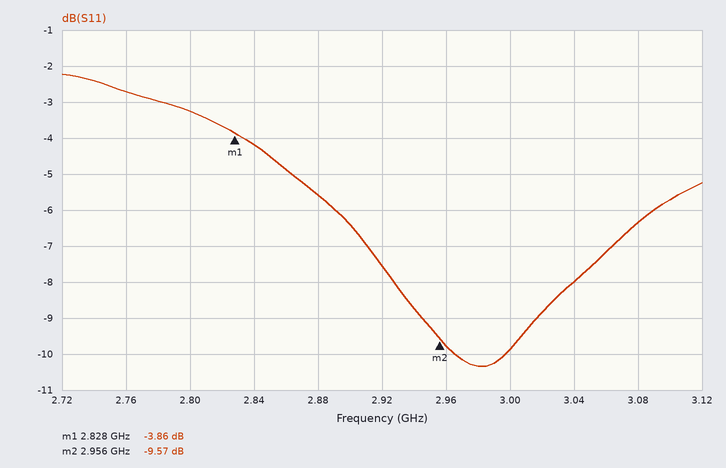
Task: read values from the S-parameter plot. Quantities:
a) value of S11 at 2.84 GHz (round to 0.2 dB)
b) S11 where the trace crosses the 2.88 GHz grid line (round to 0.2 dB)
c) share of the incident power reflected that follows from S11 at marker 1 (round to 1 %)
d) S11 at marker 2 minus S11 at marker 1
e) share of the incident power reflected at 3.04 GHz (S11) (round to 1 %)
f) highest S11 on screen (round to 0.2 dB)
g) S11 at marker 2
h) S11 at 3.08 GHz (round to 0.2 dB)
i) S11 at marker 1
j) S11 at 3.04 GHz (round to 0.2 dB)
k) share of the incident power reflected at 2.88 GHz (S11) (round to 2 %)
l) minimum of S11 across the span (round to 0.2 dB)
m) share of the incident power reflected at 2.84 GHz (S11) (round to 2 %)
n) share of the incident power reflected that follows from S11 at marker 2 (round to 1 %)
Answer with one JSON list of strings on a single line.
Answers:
["-4.2 dB", "-5.6 dB", "41 %", "-5.71 dB", "16 %", "-2.2 dB", "-9.57 dB", "-6.4 dB", "-3.86 dB", "-8.0 dB", "28 %", "-10.4 dB", "38 %", "11 %"]
